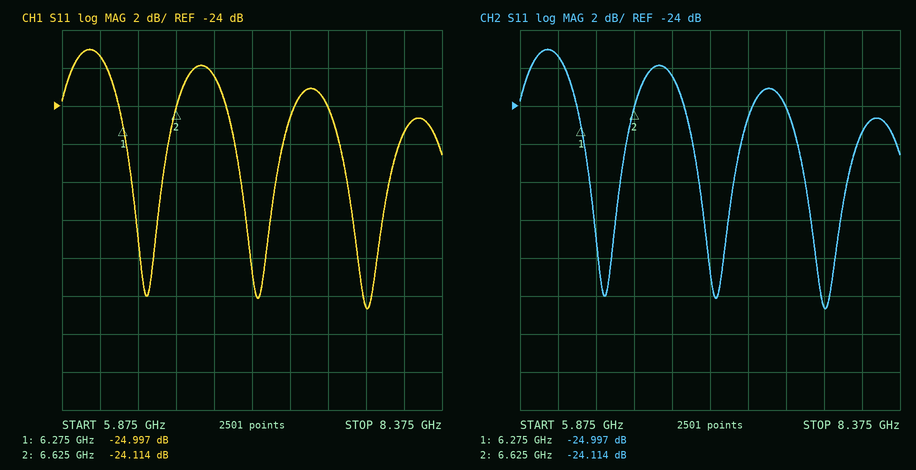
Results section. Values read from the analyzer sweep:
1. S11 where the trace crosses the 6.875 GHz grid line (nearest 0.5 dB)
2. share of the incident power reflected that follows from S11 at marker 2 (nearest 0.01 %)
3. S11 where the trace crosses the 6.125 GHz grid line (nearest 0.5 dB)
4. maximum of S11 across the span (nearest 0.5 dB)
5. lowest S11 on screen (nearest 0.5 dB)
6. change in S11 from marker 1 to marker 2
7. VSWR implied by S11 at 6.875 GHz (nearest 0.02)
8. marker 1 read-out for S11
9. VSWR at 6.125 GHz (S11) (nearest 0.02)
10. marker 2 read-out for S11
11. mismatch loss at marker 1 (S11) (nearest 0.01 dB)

-22.5 dB
0.39 %
-21.5 dB
-21.0 dB
-34.5 dB
0.883 dB
1.16
-24.997 dB
1.18
-24.114 dB
0.01 dB
